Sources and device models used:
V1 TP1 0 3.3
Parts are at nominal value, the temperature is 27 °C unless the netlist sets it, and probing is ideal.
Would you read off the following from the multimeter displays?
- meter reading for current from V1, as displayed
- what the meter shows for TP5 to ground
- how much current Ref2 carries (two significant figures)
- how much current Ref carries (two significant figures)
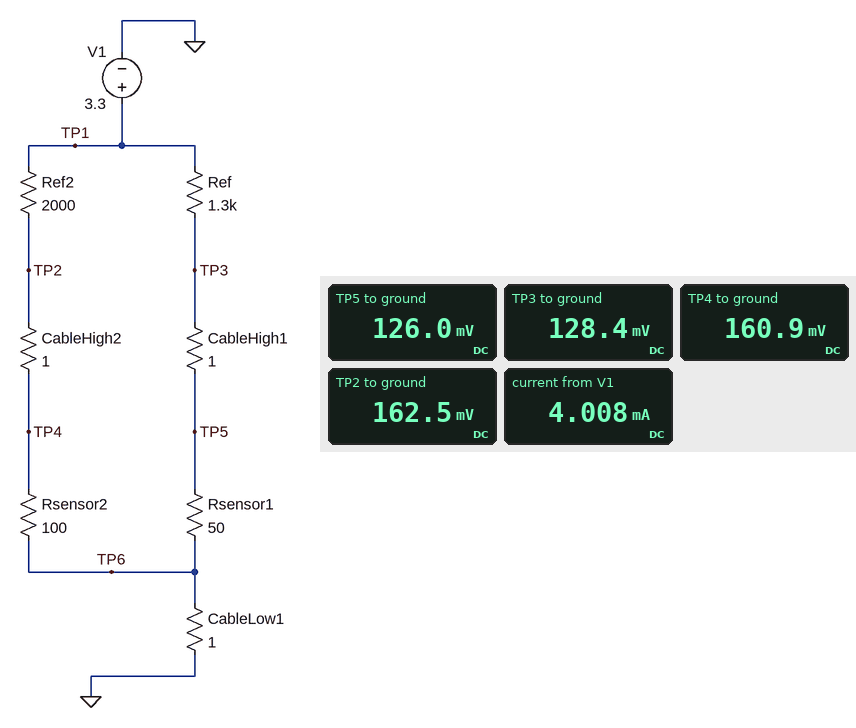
4.008 mA
126.0 mV
1.6 mA
2.4 mA
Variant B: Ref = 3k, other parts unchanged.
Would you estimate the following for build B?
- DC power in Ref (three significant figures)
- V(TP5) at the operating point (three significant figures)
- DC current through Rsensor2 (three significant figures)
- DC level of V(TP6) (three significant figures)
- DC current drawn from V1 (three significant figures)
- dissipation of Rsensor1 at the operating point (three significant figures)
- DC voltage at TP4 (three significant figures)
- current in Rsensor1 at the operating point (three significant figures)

3.50 mW
56.7 mV
1.57 mA
2.65 mV
2.65 mA
58.4 µW
160 mV
1.08 mA
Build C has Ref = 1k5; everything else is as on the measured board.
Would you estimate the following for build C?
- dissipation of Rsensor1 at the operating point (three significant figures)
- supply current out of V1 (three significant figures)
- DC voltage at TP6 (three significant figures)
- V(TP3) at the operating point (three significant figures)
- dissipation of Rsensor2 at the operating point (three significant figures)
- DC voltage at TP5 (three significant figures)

226 µW
3.69 mA
3.69 mV
112 mV
246 µW
110 mV
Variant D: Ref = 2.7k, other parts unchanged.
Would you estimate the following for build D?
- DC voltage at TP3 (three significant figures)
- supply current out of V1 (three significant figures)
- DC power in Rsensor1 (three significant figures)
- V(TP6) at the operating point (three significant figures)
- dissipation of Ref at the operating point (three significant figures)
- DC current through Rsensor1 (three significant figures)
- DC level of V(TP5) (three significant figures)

63.9 mV
2.77 mA
71.8 µW
2.77 mV
3.88 mW
1.20 mA
62.7 mV
